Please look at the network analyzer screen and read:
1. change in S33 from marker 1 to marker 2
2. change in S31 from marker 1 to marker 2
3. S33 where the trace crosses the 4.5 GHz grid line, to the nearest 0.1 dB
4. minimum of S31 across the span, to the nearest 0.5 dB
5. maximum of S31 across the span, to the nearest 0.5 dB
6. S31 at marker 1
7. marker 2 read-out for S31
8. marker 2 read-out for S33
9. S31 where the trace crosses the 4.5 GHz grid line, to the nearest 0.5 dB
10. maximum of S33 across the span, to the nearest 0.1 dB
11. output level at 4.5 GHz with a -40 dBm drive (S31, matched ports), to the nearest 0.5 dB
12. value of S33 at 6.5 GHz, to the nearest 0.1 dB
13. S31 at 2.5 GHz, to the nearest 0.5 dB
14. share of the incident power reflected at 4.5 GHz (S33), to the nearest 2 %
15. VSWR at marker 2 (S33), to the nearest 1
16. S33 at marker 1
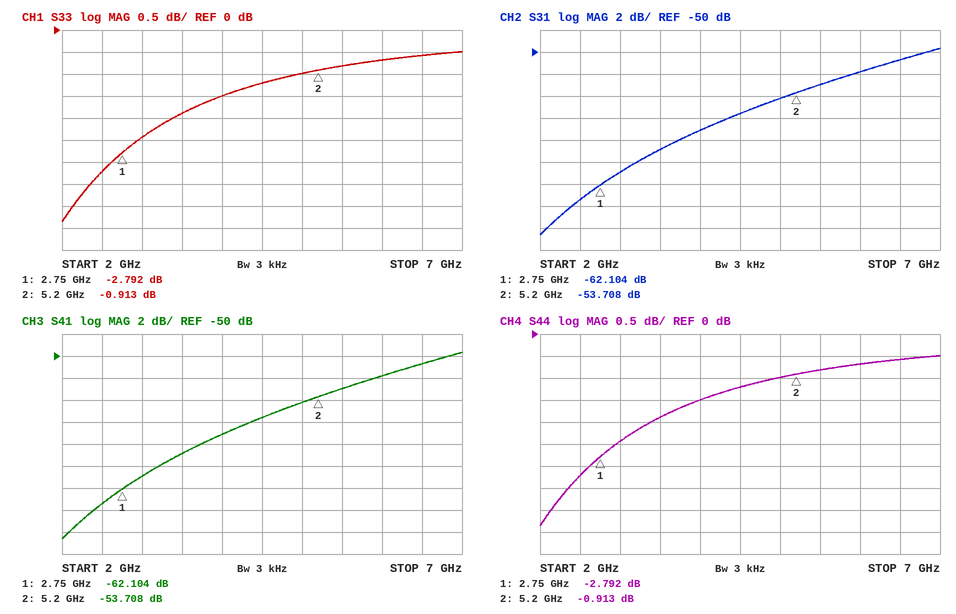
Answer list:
1.879 dB
8.396 dB
-1.2 dB
-66.5 dB
-49.5 dB
-62.104 dB
-53.708 dB
-0.913 dB
-55.5 dB
-0.5 dB
-95.5 dBm
-0.6 dB
-63.5 dB
76 %
19
-2.792 dB
